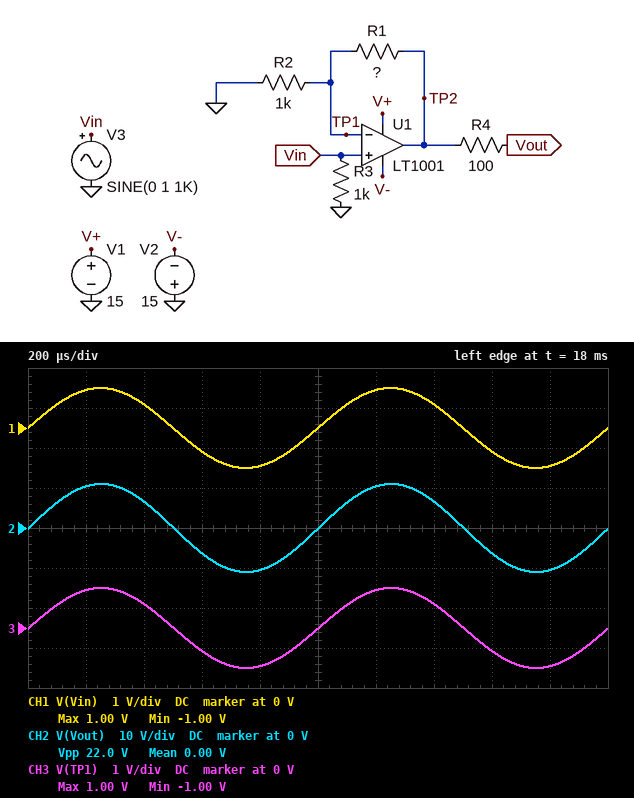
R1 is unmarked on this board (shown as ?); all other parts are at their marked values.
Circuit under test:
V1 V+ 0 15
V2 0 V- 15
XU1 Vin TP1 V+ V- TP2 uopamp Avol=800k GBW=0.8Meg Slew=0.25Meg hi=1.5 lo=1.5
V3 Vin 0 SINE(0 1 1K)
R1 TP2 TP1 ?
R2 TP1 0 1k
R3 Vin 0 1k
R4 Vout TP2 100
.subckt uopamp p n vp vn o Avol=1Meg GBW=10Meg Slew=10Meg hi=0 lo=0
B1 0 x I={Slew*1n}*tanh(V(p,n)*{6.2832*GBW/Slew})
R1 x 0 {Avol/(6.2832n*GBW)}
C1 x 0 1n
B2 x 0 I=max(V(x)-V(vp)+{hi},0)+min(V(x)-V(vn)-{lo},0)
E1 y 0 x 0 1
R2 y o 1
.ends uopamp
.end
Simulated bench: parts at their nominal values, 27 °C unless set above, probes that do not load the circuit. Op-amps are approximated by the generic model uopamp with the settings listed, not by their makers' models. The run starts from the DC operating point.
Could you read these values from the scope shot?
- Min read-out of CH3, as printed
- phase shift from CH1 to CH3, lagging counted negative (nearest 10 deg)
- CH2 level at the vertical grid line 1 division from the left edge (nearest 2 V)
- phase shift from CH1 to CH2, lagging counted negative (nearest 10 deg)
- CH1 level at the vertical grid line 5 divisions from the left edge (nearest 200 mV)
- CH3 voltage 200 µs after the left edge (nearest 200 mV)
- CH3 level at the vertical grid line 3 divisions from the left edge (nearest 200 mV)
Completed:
-1.00 V
0 deg
10 V
0 deg
0 V
1.0 V
-600 mV
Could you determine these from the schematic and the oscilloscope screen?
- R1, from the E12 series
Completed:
10 kΩ
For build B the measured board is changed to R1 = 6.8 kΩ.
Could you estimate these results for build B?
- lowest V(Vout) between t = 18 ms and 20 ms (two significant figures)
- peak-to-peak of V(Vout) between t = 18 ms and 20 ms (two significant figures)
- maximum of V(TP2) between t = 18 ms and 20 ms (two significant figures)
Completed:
-7.8 V
16 V
7.8 V
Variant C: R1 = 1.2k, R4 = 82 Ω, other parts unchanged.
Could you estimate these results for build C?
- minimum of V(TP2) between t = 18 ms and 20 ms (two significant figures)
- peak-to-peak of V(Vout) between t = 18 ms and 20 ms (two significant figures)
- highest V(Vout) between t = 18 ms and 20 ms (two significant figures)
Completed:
-2.2 V
4.4 V
2.2 V
